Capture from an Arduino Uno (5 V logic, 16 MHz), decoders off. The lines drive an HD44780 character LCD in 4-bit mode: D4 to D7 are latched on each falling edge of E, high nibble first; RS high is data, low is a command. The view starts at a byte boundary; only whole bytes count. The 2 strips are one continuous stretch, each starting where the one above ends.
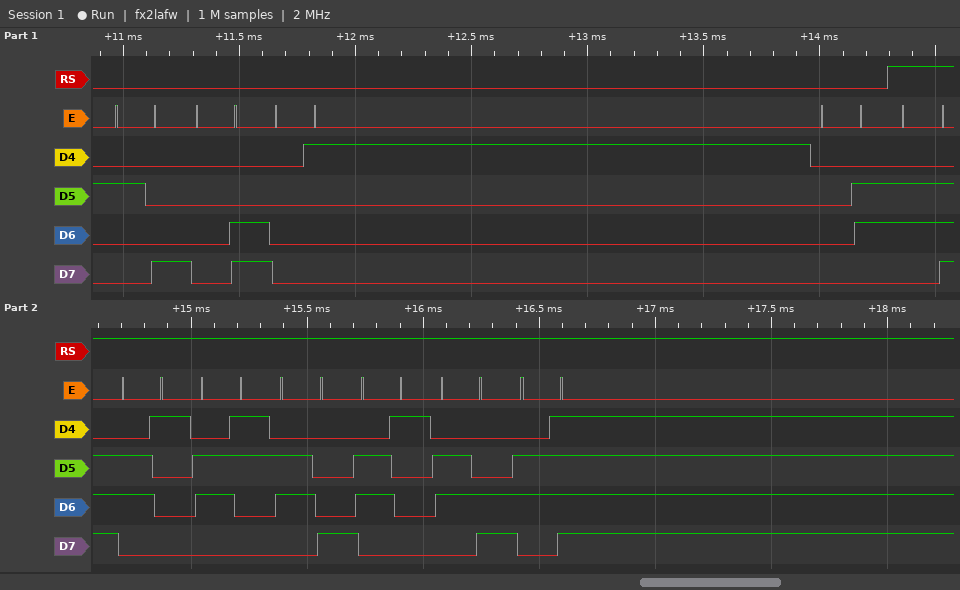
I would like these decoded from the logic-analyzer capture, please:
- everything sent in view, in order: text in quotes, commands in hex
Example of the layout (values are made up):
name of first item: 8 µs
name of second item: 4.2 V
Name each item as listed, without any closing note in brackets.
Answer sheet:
everything sent in view, in order: text in quotes, commands in hex: 0x28 0x0C 0x01 0x06 "nachalo"
